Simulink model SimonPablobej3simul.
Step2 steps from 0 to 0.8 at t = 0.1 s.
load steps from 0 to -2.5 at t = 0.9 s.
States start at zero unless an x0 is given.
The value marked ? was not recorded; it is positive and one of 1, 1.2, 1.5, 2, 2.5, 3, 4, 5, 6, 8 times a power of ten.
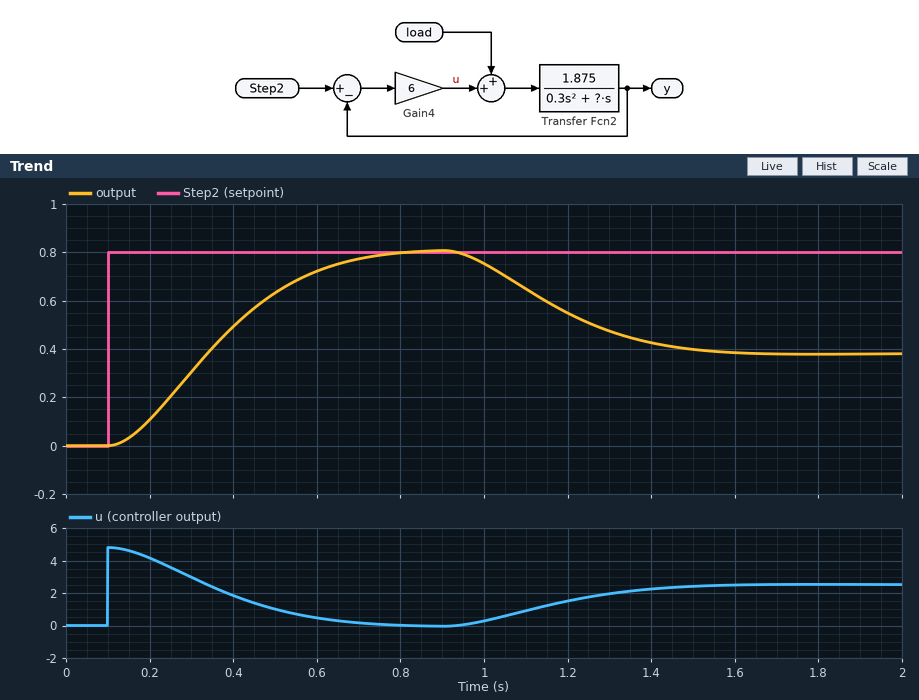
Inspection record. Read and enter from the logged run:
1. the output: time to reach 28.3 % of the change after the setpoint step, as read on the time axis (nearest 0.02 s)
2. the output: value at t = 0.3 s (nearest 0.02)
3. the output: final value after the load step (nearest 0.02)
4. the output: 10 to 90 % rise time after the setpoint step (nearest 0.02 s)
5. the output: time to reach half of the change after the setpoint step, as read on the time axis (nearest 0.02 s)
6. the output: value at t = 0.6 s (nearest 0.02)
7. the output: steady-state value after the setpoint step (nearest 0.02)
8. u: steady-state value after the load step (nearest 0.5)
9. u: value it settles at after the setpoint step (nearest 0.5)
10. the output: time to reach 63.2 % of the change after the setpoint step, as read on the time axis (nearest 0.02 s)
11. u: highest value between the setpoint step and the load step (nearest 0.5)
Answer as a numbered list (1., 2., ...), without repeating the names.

1. 0.26 s
2. 0.30
3. 0.38
4. 0.42 s
5. 0.34 s
6. 0.72
7. 0.80
8. 2.5
9. 0.0
10. 0.40 s
11. 5.0
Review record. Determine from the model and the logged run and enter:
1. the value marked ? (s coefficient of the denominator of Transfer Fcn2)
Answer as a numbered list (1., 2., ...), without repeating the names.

1. 3
